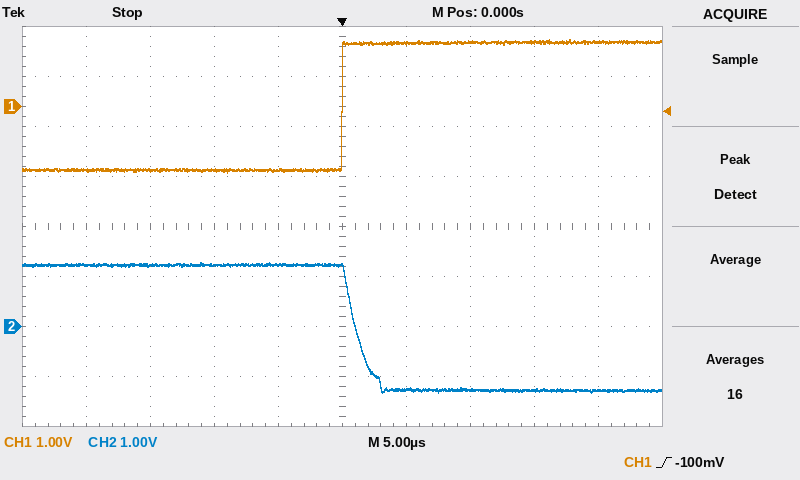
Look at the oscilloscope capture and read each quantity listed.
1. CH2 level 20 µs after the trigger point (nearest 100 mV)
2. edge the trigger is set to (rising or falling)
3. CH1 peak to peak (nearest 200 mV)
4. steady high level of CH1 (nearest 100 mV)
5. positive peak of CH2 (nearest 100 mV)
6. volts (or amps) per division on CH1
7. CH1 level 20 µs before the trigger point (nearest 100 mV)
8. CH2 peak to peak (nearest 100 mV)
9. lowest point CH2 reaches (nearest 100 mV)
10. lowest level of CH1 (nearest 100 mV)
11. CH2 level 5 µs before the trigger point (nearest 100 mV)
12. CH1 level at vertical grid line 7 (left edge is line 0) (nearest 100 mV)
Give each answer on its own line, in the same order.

-1.3 V
rising
2.6 V
1.3 V
1.3 V
1 V
-1.3 V
2.6 V
-1.3 V
-1.3 V
1.2 V
1.3 V
